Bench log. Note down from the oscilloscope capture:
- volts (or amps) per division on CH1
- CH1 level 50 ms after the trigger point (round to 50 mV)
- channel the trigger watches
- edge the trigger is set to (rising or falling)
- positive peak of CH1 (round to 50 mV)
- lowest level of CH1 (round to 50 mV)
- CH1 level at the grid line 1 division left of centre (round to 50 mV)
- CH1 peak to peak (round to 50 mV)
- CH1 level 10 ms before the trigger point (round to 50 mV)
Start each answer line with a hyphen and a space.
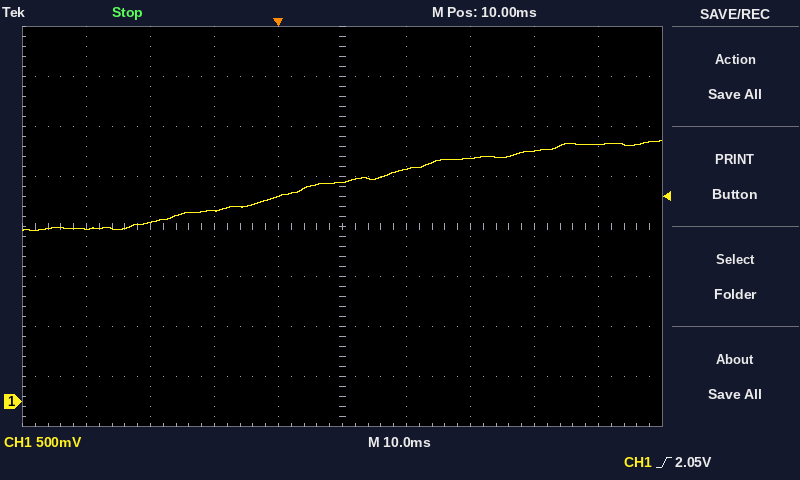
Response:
- 500 mV
- 2.55 V
- CH1
- rising
- 2.60 V
- 1.70 V
- 2.05 V
- 900 mV
- 1.90 V
